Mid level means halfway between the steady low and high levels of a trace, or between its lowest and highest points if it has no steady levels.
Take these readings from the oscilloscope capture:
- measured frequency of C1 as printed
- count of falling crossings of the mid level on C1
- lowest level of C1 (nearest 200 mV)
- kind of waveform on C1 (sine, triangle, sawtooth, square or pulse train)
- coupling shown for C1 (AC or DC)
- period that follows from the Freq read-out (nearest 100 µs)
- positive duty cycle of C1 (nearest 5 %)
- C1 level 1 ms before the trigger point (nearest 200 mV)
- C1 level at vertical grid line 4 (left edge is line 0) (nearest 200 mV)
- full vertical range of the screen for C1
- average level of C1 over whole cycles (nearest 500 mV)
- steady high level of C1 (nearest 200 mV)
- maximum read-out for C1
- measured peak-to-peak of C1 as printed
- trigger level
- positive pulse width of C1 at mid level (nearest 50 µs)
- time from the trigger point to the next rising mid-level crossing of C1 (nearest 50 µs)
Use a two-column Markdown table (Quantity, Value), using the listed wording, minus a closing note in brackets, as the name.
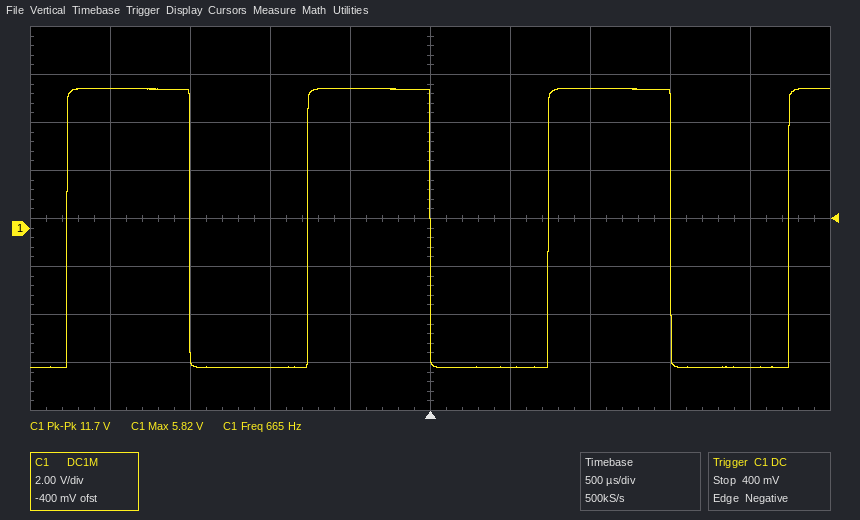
| Quantity | Value |
|---|---|
| measured frequency of C1 as printed | 665 Hz |
| count of falling crossings of the mid level on C1 | 3 |
| lowest level of C1 | -5.8 V |
| kind of waveform on C1 | square |
| coupling shown for C1 | DC |
| period that follows from the Freq read-out | 1.5 ms |
| positive duty cycle of C1 | 50 % |
| C1 level 1 ms before the trigger point | -5.8 V |
| C1 level at vertical grid line 4 (left edge is line 0) | 5.8 V |
| full vertical range of the screen for C1 | 16 V |
| average level of C1 over whole cycles | 0.0 V |
| steady high level of C1 | 5.8 V |
| maximum read-out for C1 | 5.82 V |
| measured peak-to-peak of C1 as printed | 11.7 V |
| trigger level | 400 mV |
| positive pulse width of C1 at mid level | 750 µs |
| time from the trigger point to the next rising mid-level crossing of C1 | 750 µs |
